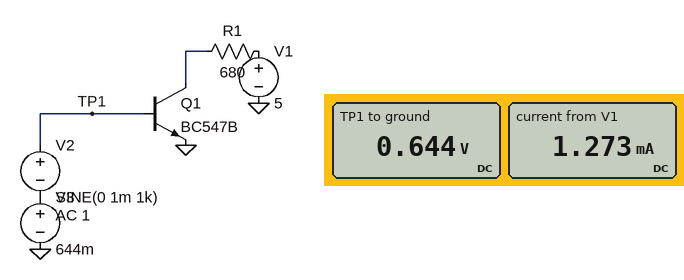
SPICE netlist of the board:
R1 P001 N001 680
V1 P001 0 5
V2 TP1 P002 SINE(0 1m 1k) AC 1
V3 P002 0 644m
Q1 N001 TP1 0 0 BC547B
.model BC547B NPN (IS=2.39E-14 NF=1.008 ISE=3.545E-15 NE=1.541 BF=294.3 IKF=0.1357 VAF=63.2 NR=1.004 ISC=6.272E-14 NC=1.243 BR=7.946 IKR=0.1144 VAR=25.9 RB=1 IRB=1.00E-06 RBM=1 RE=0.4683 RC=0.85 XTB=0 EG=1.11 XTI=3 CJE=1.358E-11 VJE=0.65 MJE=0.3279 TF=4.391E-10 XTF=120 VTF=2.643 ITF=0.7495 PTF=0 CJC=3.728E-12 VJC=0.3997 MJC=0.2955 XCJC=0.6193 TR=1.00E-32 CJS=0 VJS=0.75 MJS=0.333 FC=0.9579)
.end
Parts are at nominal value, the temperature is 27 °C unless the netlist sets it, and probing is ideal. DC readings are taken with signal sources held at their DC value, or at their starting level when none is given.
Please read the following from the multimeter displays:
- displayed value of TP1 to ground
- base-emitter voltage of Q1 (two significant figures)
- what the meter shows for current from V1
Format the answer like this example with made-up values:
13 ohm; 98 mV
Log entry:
0.644 V; 640 mV; 1.273 mA
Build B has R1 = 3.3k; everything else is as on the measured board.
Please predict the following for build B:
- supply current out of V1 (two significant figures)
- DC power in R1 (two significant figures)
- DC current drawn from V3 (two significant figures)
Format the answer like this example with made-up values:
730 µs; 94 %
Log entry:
1.2 mA; 4.9 mW; 4.3 µA
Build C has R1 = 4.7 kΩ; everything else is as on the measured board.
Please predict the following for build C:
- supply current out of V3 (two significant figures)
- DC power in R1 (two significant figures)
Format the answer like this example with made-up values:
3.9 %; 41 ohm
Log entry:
25 µA; 5.2 mW
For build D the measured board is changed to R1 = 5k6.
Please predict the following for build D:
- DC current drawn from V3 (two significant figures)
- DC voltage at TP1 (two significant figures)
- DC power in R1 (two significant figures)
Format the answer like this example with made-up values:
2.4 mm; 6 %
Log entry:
48 µA; 640 mV; 4.4 mW
